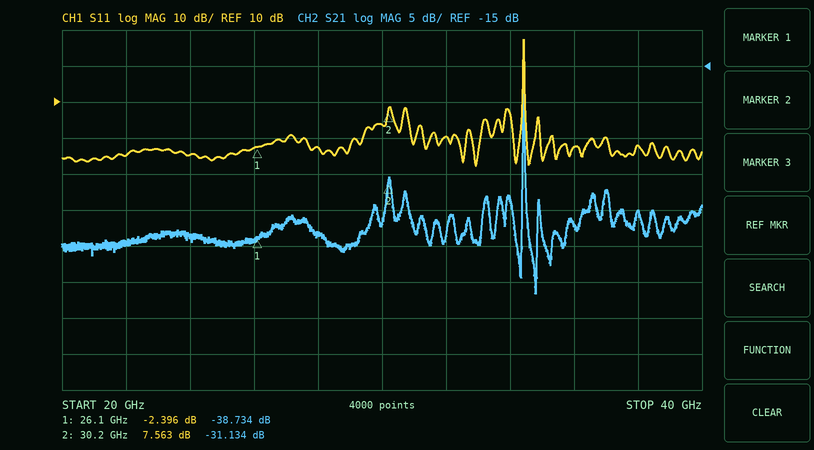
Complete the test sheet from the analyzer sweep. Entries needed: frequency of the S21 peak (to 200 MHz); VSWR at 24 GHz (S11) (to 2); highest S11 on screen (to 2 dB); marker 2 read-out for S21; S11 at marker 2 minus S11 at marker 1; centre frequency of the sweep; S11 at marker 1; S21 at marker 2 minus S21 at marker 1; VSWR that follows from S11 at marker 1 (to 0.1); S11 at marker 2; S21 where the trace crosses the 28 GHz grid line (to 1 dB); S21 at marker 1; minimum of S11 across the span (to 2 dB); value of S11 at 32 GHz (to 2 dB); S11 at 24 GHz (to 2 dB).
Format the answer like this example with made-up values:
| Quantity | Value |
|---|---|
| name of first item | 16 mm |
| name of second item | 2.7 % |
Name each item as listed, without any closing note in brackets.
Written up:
| Quantity | Value |
|---|---|
| frequency of the S21 peak | 34.4 GHz |
| VSWR at 24 GHz (S11) | 4 |
| highest S11 on screen | 28 dB |
| marker 2 read-out for S21 | -31.134 dB |
| S11 at marker 2 minus S11 at marker 1 | 9.959 dB |
| centre frequency of the sweep | 30 GHz |
| S11 at marker 1 | -2.396 dB |
| S21 at marker 2 minus S21 at marker 1 | 7.600 dB |
| VSWR that follows from S11 at marker 1 | 7.3 |
| S11 at marker 2 | 7.563 dB |
| S21 where the trace crosses the 28 GHz grid line | -38 dB |
| S21 at marker 1 | -38.734 dB |
| minimum of S11 across the span | -8 dB |
| value of S11 at 32 GHz | 0 dB |
| S11 at 24 GHz | -4 dB |
